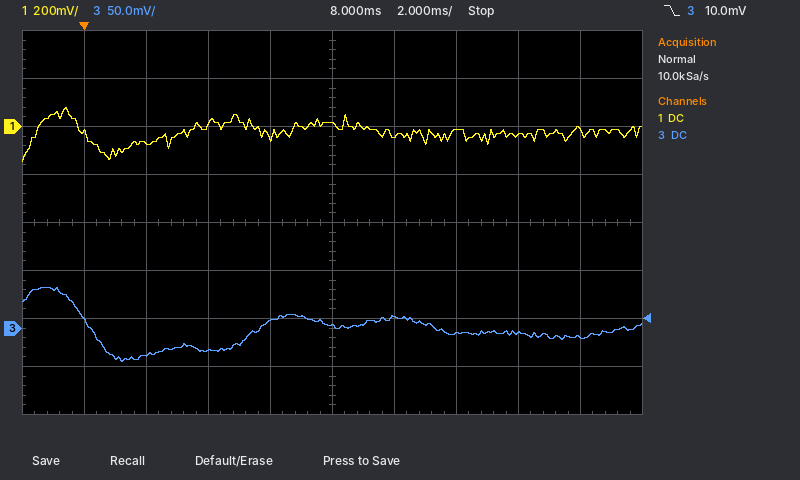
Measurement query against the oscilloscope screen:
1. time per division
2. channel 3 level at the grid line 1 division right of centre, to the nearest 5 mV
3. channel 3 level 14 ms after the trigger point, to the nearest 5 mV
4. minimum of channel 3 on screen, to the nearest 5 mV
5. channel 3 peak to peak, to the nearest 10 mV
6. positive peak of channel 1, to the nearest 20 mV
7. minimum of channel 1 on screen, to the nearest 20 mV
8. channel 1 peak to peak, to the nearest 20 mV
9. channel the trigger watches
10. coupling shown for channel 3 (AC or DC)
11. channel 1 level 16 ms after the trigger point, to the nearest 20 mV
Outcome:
2 ms
10 mV
-5 mV
-35 mV
80 mV
80 mV
-140 mV
220 mV
channel 3
DC
-20 mV
